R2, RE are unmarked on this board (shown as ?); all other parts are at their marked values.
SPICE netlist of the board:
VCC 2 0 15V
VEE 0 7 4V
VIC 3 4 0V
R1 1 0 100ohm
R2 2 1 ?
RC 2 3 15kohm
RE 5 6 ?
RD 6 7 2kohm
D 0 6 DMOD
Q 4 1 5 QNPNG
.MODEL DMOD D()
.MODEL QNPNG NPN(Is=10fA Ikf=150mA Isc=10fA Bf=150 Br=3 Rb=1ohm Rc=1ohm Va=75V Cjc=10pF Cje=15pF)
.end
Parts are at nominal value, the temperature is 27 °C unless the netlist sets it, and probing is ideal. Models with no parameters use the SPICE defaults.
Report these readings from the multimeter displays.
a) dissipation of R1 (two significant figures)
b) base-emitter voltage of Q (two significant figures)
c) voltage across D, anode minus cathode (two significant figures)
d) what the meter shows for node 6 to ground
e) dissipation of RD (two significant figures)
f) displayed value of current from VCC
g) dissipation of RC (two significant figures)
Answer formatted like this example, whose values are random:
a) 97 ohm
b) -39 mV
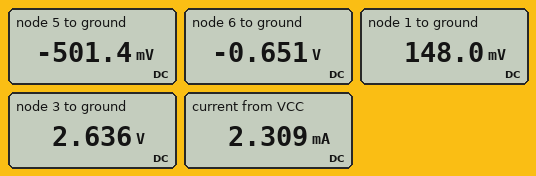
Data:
a) 220 µW
b) 650 mV
c) 650 mV
d) -0.651 V
e) 5.6 mW
f) 2.309 mA
g) 10 mW
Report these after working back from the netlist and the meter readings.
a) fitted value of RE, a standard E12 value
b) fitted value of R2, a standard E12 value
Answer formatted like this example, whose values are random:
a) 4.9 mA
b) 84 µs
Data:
a) 180 Ω
b) 10 kΩ
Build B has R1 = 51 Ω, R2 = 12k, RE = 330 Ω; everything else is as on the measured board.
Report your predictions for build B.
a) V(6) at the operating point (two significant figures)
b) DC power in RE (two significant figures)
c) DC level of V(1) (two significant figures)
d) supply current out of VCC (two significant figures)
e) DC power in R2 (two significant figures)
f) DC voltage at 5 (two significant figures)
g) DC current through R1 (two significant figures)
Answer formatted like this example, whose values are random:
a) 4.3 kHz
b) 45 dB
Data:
a) -660 mV
b) 33 µW
c) 63 mV
d) 1.6 mA
e) 19 mW
f) -560 mV
g) 1.2 mA
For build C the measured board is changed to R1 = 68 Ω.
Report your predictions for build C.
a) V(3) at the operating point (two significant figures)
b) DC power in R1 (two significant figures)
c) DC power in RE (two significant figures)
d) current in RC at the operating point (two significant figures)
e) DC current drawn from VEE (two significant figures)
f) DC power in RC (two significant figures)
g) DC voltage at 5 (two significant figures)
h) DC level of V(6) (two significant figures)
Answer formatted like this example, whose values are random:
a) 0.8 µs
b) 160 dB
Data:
a) 5.5 V
b) 150 µW
c) 74 µW
d) 640 µA
e) 1.7 mA
f) 6.1 mW
g) -540 mV
h) -660 mV
